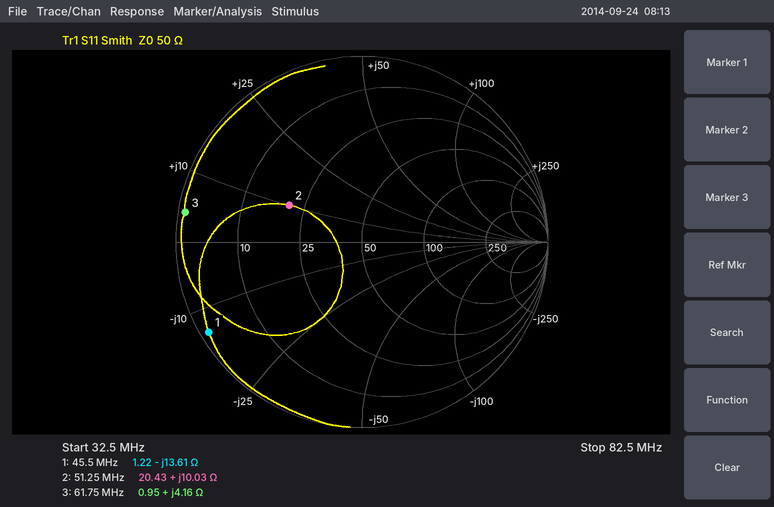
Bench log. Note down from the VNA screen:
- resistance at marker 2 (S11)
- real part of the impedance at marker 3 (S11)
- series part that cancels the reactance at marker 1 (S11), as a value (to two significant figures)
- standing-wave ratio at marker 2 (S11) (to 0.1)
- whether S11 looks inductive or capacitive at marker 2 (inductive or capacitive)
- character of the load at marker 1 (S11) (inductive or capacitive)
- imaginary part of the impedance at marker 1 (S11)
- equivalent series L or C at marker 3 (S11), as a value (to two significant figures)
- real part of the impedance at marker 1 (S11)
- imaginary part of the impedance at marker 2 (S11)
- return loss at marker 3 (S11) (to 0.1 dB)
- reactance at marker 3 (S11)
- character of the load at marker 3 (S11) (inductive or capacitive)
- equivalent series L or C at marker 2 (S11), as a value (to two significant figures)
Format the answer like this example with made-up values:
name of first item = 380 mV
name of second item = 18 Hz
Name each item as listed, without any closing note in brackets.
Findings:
resistance at marker 2 = 20.43 Ω
real part of the impedance at marker 3 = 0.95 Ω
series part that cancels the reactance at marker 1 (S11), as a value = 48 nH
standing-wave ratio at marker 2 (S11) = 2.6
whether S11 looks inductive or capacitive at marker 2 = inductive
character of the load at marker 1 (S11) = capacitive
imaginary part of the impedance at marker 1 = -13.61 Ω
equivalent series L or C at marker 3 (S11), as a value = 11 nH
real part of the impedance at marker 1 = 1.22 Ω
imaginary part of the impedance at marker 2 = +10.03 Ω
return loss at marker 3 (S11) = 0.3 dB
reactance at marker 3 = +4.16 Ω
character of the load at marker 3 (S11) = inductive
equivalent series L or C at marker 2 (S11), as a value = 31 nH
